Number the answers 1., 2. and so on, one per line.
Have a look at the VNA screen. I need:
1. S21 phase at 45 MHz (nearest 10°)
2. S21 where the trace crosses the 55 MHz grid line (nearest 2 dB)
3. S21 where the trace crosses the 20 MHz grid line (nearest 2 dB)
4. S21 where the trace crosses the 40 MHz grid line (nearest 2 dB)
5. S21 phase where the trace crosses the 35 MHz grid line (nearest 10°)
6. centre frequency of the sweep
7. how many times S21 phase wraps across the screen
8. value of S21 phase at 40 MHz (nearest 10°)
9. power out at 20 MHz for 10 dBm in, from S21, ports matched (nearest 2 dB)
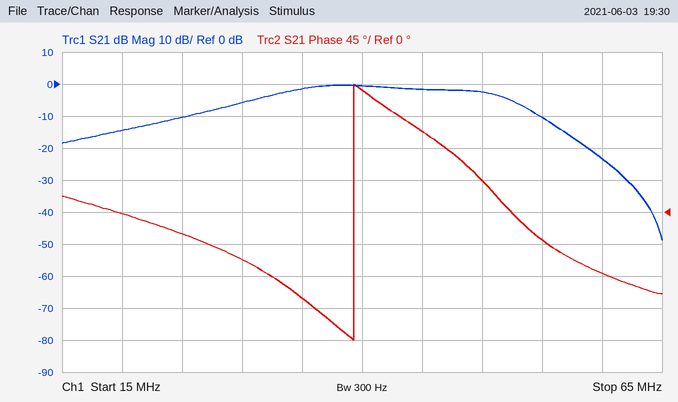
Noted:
1. 110°
2. -10 dB
3. -14 dB
4. 0 dB
5. -120°
6. 40 MHz
7. 1
8. 170°
9. -4 dBm
